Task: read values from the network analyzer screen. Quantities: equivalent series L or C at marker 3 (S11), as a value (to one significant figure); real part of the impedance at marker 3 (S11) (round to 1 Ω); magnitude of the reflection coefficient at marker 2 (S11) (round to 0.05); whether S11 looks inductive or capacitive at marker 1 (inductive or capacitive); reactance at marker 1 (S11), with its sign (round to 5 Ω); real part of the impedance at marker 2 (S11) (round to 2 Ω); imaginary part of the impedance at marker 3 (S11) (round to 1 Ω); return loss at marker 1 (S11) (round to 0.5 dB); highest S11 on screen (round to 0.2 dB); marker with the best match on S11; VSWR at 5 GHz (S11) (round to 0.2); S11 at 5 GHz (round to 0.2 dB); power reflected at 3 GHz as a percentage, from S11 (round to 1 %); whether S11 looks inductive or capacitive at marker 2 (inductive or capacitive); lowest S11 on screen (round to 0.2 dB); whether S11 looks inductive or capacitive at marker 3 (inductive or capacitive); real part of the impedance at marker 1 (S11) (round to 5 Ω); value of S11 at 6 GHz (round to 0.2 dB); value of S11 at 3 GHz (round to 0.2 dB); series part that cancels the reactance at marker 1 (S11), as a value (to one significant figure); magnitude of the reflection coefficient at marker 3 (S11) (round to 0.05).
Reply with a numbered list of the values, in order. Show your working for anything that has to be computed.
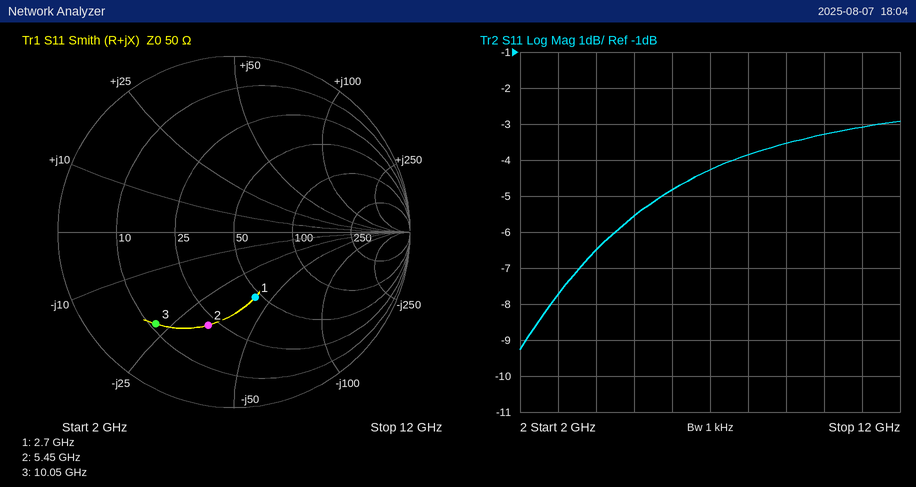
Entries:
1. C = 1/(2π × 10.05 GHz × 22 Ω) ≈ 720 fF, so 700 fF to one significant figure
2. 11 Ω
3. 0.55
4. capacitive
5. -40 Ω
6. 22 Ω
7. -22 Ω
8. 8.0 dB
9. -3.0 dB
10. marker 1
11. |Γ| = 10^(-5.6/20) = 0.5248; VSWR = (1 + 0.5248)/(1 − 0.5248) ≈ 3.2
12. -5.6 dB
13. 10^(-7.8/10) ≈ 17 %
14. capacitive
15. -9.2 dB
16. capacitive
17. 45 Ω
18. -4.8 dB
19. -7.8 dB
20. L = 40 Ω/(2π × 2.7 GHz) ≈ 2 nH
21. 0.70
